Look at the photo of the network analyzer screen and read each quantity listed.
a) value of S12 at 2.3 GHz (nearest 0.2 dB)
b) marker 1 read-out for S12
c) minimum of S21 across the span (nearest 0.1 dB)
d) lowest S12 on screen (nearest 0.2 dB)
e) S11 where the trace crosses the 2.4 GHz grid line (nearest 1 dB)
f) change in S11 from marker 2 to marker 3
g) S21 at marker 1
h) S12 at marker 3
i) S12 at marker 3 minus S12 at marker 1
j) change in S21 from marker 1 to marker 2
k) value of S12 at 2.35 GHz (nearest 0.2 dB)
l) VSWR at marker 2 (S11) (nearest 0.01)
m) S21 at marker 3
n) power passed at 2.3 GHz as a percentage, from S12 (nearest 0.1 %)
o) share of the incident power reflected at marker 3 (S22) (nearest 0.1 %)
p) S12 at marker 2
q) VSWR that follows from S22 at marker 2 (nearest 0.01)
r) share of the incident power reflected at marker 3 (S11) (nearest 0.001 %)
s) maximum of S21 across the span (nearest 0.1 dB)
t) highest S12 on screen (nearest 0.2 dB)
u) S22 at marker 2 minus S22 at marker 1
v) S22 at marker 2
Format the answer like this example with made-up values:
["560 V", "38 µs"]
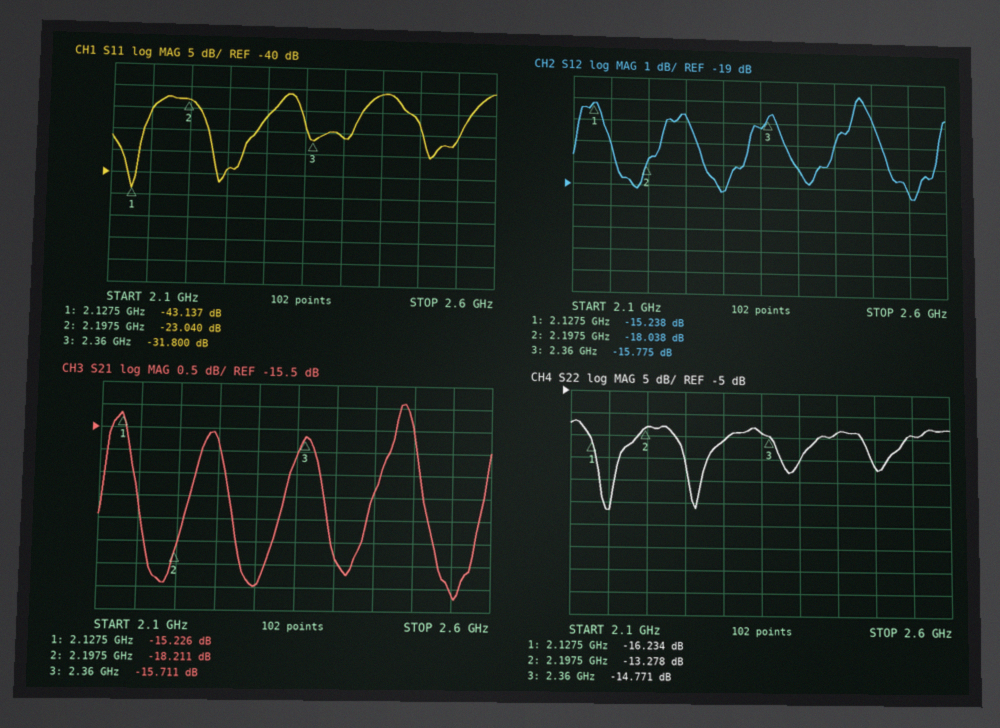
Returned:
["-19.2 dB", "-15.238 dB", "-19.2 dB", "-19.4 dB", "-31 dB", "-8.760 dB", "-15.226 dB", "-15.775 dB", "-0.537 dB", "-2.985 dB", "-16.2 dB", "1.15", "-15.711 dB", "1.2 %", "3.3 %", "-18.038 dB", "1.55", "0.066 %", "-14.9 dB", "-14.6 dB", "2.956 dB", "-13.278 dB"]
